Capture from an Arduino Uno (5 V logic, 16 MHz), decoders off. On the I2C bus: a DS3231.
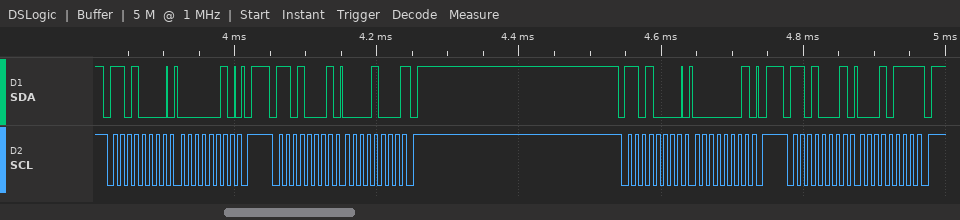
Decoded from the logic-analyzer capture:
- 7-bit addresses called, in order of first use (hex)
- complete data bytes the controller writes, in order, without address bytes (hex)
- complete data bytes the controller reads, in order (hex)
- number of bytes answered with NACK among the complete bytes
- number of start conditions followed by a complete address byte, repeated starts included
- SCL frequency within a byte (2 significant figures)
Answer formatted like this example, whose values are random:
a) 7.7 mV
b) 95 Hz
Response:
a) 0x68
b) 02 01
c) 08 17
d) 2
e) 4
f) 100 kHz
